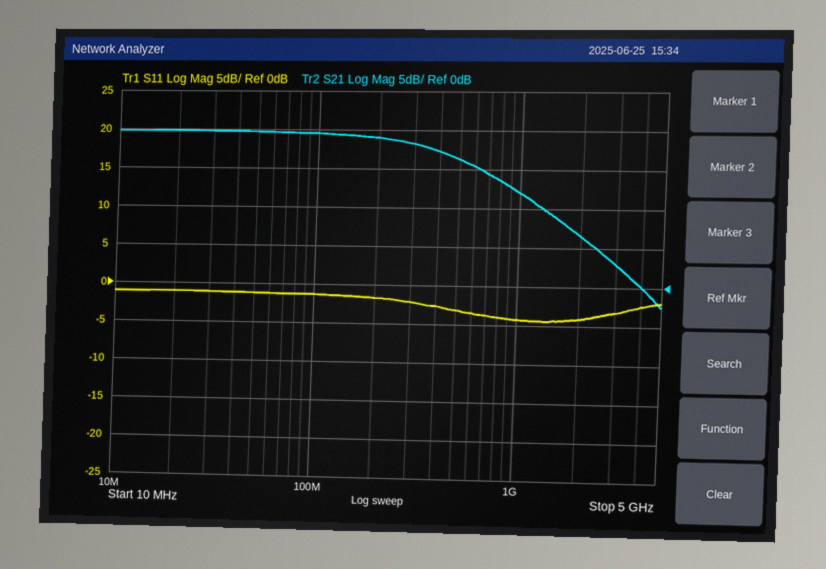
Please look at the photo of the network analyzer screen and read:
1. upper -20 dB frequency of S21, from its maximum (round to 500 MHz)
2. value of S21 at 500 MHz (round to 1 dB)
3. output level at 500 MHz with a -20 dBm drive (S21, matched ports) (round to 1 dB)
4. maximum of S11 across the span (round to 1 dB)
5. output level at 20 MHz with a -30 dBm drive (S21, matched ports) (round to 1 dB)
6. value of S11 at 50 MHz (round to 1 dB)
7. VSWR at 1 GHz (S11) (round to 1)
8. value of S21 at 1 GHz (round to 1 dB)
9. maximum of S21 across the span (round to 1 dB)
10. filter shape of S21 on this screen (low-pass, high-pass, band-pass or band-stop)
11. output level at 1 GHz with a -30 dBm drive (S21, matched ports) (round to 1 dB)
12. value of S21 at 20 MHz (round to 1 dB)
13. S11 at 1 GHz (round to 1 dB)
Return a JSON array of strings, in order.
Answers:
["4.0 GHz", "16 dB", "-4 dBm", "-1 dB", "-10 dBm", "-1 dB", "4", "12 dB", "20 dB", "low-pass", "-18 dBm", "20 dB", "-4 dB"]
